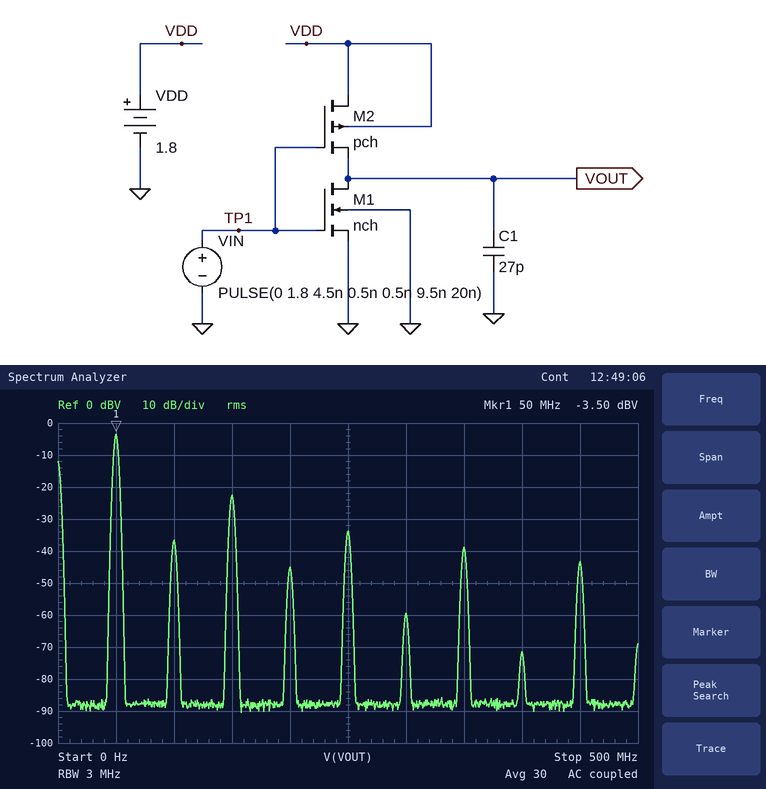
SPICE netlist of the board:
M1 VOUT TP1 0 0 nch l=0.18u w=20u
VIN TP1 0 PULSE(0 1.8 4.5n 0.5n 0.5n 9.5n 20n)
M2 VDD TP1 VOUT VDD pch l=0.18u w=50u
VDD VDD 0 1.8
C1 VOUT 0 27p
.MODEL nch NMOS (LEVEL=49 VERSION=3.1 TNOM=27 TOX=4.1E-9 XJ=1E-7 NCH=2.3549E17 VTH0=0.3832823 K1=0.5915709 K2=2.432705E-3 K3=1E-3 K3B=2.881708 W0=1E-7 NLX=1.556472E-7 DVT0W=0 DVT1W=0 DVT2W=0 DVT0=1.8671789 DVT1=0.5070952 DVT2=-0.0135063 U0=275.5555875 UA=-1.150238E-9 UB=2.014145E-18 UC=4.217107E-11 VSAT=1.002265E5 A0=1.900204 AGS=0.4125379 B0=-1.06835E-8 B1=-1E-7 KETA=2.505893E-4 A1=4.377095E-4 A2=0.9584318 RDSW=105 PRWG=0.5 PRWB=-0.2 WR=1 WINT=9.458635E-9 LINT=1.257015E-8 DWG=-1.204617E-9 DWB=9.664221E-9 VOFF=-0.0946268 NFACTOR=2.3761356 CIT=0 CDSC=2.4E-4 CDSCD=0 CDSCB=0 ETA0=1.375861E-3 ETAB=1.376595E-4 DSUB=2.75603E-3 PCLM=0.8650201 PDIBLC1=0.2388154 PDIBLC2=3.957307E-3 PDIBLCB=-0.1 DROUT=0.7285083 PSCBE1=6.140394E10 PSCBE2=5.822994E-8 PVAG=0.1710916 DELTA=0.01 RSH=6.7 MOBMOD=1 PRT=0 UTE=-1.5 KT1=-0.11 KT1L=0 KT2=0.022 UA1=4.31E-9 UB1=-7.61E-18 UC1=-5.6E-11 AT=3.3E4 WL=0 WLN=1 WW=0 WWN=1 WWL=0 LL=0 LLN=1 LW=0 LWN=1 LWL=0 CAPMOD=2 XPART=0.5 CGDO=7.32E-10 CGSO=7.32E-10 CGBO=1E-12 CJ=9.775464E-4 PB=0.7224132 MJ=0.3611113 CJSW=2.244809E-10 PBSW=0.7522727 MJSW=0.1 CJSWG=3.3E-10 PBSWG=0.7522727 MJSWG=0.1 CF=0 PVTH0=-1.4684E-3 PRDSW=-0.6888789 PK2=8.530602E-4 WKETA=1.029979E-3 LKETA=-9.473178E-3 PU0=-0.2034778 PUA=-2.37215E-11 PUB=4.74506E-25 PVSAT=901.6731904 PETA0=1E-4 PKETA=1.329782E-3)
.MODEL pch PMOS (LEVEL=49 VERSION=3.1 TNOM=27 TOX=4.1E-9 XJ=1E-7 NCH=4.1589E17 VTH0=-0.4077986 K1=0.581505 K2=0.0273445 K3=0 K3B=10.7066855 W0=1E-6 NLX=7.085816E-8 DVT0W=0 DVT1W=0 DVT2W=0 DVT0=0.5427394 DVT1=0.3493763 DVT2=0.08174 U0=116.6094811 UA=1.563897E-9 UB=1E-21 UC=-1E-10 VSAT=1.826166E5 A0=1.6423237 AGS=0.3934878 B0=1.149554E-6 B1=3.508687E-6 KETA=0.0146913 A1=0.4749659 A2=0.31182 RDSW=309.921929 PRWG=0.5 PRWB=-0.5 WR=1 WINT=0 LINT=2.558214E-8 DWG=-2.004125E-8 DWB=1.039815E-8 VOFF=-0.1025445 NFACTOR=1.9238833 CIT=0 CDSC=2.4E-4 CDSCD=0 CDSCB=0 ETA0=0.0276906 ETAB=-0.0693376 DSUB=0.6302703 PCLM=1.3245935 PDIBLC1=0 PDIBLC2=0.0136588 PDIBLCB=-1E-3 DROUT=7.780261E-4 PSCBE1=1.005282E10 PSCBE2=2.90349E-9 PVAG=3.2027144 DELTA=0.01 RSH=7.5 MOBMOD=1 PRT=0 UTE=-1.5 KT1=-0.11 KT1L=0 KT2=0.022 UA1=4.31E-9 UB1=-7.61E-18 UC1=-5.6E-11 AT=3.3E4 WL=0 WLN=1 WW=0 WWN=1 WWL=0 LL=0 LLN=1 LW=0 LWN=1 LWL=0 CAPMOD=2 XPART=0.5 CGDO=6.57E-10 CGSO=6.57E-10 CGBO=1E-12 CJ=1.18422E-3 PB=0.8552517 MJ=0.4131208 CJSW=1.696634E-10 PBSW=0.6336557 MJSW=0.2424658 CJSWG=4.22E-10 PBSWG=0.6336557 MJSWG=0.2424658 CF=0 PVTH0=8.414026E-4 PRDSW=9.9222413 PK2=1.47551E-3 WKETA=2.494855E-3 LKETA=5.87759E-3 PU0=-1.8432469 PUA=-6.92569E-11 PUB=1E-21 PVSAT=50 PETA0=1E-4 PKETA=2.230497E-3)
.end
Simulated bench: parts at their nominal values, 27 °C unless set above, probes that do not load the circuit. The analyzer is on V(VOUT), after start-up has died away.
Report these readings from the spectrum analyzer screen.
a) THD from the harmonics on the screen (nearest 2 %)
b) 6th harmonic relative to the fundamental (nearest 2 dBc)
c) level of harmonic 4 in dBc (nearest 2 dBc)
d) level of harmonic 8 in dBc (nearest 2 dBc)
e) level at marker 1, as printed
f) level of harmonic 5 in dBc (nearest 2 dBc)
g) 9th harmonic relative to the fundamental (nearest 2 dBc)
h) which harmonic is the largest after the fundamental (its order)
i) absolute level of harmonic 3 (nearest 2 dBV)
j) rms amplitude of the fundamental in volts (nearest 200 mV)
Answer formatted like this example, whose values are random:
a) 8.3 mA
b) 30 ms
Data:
a) 12 %
b) -56 dBc
c) -42 dBc
d) -68 dBc
e) -3.50 dBV
f) -30 dBc
g) -40 dBc
h) 3
i) -22 dBV
j) 600 mV
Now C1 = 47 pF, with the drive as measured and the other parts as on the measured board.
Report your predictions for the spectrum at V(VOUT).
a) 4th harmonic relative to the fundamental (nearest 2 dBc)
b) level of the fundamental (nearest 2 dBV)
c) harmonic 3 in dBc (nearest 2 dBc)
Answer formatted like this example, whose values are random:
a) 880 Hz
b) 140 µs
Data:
a) -54 dBc
b) -6 dBV
c) -22 dBc
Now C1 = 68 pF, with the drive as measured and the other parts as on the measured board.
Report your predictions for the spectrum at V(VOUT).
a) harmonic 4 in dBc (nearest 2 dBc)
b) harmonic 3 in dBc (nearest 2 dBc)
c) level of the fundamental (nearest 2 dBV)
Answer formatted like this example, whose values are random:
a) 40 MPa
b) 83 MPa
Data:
a) -52 dBc
b) -20 dBc
c) -8 dBV
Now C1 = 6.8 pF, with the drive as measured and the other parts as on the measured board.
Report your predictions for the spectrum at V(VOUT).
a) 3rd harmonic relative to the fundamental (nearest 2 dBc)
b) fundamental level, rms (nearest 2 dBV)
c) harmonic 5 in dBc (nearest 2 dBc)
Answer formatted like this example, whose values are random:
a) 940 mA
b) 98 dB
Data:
a) -10 dBc
b) -2 dBV
c) -16 dBc
